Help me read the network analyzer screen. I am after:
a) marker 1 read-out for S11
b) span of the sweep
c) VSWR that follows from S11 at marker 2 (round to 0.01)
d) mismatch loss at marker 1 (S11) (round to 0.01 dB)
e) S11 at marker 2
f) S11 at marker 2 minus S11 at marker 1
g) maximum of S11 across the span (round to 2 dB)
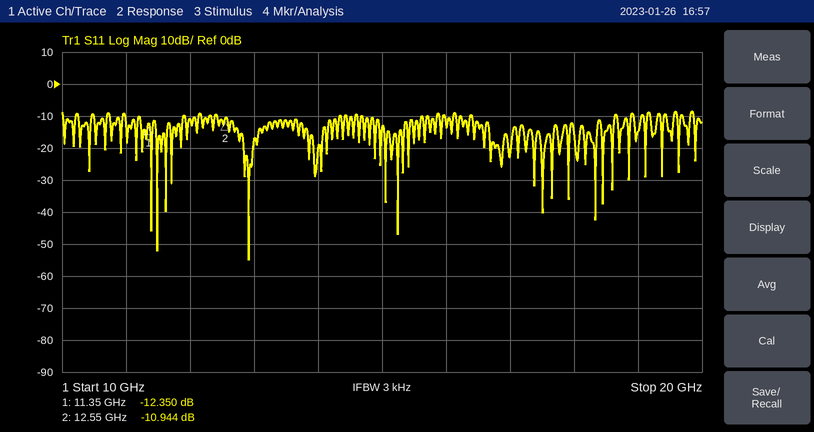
-12.350 dB
10 GHz
1.79
0.26 dB
-10.944 dB
1.406 dB
-8 dB
